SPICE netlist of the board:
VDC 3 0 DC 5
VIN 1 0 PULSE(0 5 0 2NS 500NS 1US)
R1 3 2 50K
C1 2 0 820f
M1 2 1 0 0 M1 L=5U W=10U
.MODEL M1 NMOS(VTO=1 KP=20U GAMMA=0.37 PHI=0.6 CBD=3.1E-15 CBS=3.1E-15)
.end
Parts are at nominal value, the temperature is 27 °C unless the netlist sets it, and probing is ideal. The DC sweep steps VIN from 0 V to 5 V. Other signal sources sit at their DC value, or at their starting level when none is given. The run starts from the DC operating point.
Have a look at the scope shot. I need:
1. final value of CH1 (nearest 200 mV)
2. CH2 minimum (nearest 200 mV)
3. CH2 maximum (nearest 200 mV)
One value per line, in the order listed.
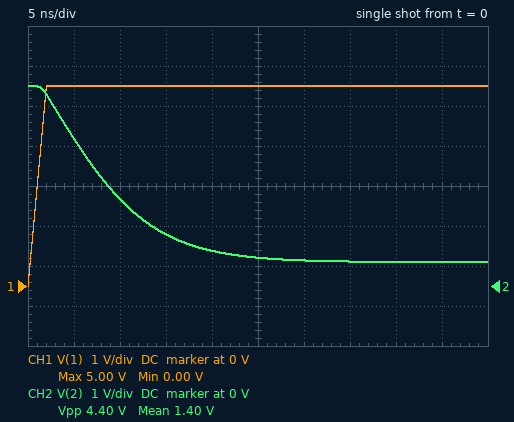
5.0 V
600 mV
5.0 V
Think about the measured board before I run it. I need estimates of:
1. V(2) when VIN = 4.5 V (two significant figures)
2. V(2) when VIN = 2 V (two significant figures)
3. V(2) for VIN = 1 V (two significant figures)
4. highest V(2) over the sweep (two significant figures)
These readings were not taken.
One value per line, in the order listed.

680 mV
4.0 V
5.0 V
5.0 V
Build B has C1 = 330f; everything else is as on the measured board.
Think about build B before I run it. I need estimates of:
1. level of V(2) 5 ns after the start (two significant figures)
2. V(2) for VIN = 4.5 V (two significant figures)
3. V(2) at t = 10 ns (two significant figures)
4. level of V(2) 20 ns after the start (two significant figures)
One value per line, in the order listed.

2.1 V
680 mV
770 mV
600 mV
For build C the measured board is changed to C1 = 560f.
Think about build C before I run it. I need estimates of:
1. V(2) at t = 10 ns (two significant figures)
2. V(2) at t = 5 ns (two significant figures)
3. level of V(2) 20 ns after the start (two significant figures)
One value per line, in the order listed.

1.4 V
3.1 V
650 mV
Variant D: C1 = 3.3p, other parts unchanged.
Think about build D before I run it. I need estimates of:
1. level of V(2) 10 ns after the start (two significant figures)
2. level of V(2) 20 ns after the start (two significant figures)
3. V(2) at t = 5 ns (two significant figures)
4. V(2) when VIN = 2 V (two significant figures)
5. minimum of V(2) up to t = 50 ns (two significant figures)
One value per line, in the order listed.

4.2 V
3.3 V
4.7 V
4.0 V
1.5 V
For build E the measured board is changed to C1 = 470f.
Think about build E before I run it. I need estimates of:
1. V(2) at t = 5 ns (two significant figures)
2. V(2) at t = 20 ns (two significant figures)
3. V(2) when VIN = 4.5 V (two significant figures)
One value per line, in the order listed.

2.8 V
620 mV
680 mV
